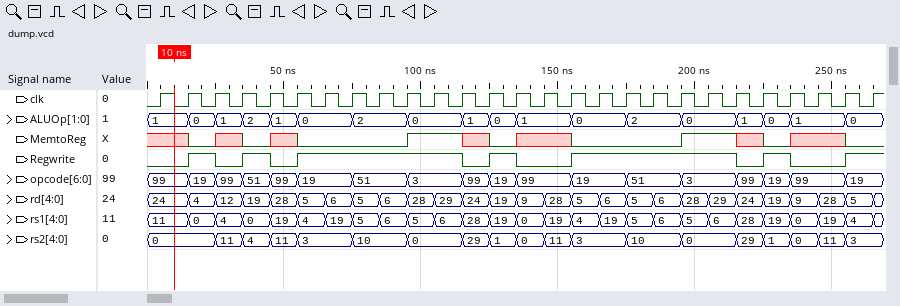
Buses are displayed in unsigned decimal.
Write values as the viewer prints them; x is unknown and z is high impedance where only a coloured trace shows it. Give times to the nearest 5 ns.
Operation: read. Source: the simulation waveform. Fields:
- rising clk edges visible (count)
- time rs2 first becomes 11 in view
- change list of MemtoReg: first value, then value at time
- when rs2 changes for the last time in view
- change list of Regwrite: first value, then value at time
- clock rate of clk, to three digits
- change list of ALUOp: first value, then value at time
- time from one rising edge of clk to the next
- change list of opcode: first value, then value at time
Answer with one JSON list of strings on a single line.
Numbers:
["27", "25 ns", "x, 0 at 15 ns, x at 25 ns, 0 at 35 ns, x at 45 ns, 0 at 55 ns, 1 at 95 ns, x at 115 ns, 0 at 125 ns, x at 135 ns, 0 at 155 ns, 1 at 195 ns, x at 215 ns, 0 at 225 ns, x at 235 ns, 0 at 255 ns", "255 ns", "0, 1 at 15 ns, 0 at 25 ns, 1 at 35 ns, 0 at 45 ns, 1 at 55 ns, 0 at 115 ns, 1 at 125 ns, 0 at 135 ns, 1 at 155 ns, 0 at 215 ns, 1 at 225 ns, 0 at 235 ns, 1 at 255 ns", "100 MHz", "1, 0 at 15 ns, 1 at 25 ns, 2 at 35 ns, 1 at 45 ns, 0 at 55 ns, 2 at 75 ns, 0 at 95 ns, 1 at 115 ns, 0 at 125 ns, 1 at 135 ns, 0 at 155 ns, 2 at 175 ns, 0 at 195 ns, 1 at 215 ns, 0 at 225 ns, 1 at 235 ns, 0 at 255 ns", "10 ns", "99, 19 at 15 ns, 99 at 25 ns, 51 at 35 ns, 99 at 45 ns, 19 at 55 ns, 51 at 75 ns, 3 at 95 ns, 99 at 115 ns, 19 at 125 ns, 99 at 135 ns, 19 at 155 ns, 51 at 175 ns, 3 at 195 ns, 99 at 215 ns, 19 at 225 ns, 99 at 235 ns, 19 at 255 ns"]
